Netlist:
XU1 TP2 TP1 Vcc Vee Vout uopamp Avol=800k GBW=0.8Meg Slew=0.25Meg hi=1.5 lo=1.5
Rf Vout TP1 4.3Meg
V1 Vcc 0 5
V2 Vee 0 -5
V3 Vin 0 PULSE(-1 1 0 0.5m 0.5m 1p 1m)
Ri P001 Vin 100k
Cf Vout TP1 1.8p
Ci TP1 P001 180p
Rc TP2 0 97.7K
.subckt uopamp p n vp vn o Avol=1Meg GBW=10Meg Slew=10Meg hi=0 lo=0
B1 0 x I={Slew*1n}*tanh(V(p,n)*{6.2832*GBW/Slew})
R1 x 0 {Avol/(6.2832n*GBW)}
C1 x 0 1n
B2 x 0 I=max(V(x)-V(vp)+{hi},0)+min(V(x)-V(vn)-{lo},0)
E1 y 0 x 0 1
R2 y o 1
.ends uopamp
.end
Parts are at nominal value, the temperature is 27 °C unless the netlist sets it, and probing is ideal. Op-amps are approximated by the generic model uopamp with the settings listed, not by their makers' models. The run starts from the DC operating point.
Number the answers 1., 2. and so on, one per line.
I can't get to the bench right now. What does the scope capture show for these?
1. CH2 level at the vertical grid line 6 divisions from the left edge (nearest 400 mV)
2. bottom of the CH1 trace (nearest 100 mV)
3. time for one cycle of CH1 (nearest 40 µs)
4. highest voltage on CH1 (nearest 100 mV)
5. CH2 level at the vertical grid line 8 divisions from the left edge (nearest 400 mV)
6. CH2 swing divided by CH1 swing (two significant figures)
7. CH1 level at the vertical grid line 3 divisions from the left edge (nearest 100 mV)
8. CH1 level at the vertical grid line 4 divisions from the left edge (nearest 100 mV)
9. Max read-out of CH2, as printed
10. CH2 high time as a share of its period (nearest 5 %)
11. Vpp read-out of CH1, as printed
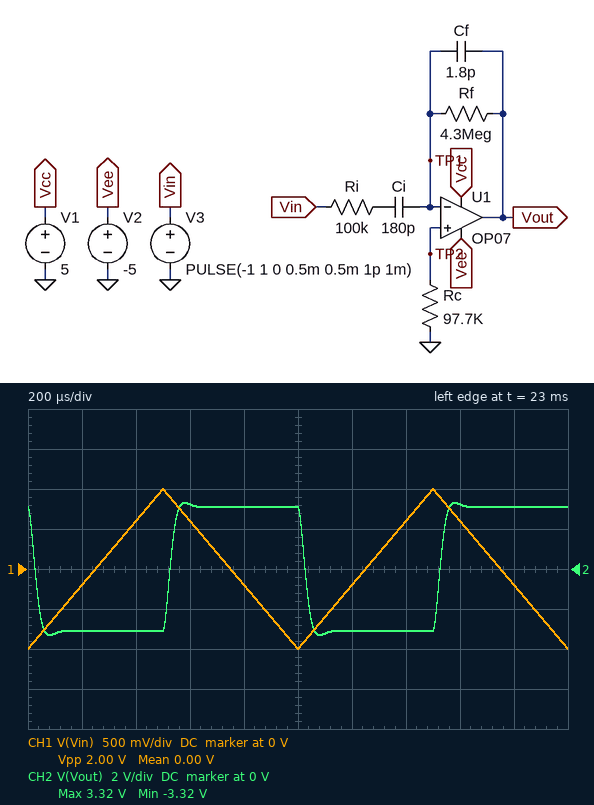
1. -3.2 V
2. -1.0 V
3. 1.00 ms
4. 1.0 V
5. 3.2 V
6. 3.3
7. 600 mV
8. -200 mV
9. 3.32 V
10. 50 %
11. 2.00 V
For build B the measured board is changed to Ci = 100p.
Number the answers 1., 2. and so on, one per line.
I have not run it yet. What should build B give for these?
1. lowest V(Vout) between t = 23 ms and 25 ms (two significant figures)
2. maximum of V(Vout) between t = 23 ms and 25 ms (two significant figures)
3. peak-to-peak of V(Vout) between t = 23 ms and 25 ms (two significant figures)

1. -1.9 V
2. 1.9 V
3. 3.8 V
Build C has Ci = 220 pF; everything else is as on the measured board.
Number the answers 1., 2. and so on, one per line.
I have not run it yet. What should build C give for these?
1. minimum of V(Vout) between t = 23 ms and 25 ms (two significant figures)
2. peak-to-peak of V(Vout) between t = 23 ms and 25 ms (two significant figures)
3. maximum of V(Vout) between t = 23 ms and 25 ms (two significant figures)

1. -3.5 V
2. 7.0 V
3. 3.5 V
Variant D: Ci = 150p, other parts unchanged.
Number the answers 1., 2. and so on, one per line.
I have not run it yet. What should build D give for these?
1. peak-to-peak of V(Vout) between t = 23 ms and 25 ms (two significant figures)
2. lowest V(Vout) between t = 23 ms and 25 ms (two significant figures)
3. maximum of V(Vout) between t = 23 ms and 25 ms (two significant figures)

1. 5.6 V
2. -2.8 V
3. 2.8 V
